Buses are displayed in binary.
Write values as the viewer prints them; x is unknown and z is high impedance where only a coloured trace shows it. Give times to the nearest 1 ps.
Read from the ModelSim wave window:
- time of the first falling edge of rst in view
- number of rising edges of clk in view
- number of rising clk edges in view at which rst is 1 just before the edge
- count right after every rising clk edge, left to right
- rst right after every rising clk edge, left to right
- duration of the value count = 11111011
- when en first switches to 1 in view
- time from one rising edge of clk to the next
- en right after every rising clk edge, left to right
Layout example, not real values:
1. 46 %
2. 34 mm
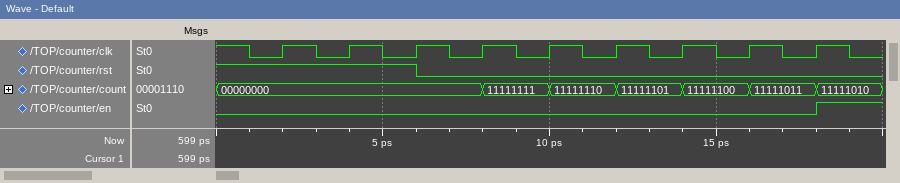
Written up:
1. 6 ps
2. 9
3. 3
4. 00000000, 00000000, 00000000, 11111111, 11111110, 11111101, 11111100, 11111011, 11111010
5. 1 1 0 0 0 0 0 0 0
6. 2 ps
7. 18 ps
8. 2 ps
9. 0 0 0 0 0 0 0 0 1
